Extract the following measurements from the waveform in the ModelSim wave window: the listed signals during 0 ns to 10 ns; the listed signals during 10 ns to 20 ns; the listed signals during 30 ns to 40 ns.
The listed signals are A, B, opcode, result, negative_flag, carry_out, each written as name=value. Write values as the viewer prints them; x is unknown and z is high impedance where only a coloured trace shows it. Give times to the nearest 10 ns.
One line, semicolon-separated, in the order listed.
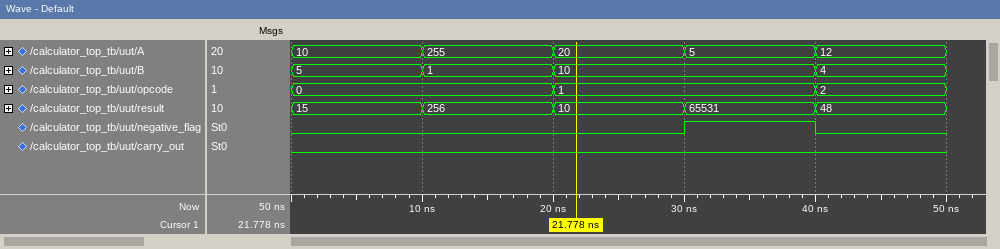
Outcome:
A=10, B=5, opcode=0, result=15, negative_flag=0, carry_out=0; A=255, B=1, opcode=0, result=256, negative_flag=0, carry_out=0; A=5, B=10, opcode=1, result=65531, negative_flag=1, carry_out=0
